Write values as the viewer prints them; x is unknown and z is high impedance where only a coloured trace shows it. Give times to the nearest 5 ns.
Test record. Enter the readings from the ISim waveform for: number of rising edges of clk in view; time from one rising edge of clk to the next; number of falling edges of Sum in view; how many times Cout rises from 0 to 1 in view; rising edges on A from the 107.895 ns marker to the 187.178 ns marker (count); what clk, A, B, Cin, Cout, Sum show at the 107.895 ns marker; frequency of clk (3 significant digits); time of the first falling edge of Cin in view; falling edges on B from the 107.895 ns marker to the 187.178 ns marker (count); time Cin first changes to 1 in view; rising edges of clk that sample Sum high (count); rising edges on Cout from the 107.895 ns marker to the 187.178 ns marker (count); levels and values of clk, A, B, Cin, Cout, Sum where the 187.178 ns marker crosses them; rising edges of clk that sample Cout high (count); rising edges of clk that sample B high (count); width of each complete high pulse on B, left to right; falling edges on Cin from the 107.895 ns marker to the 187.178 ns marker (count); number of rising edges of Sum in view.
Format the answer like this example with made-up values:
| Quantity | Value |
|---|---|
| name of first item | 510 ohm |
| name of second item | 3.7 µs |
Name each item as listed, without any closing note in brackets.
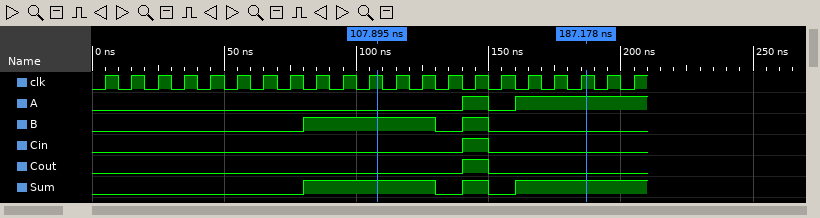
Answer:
| Quantity | Value |
|---|---|
| number of rising edges of clk in view | 21 |
| time from one rising edge of clk to the next | 10 ns |
| number of falling edges of Sum in view | 2 |
| how many times Cout rises from 0 to 1 in view | 1 |
| rising edges on A from the 107.895 ns marker to the 187.178 ns marker | 2 |
| what clk, A, B, Cin, Cout, Sum show at the 107.895 ns marker | clk=1, A=0, B=1, Cin=0, Cout=0, Sum=1 |
| frequency of clk | 100 MHz |
| time of the first falling edge of Cin in view | 150 ns |
| falling edges on B from the 107.895 ns marker to the 187.178 ns marker | 2 |
| time Cin first changes to 1 in view | 140 ns |
| rising edges of clk that sample Sum high | 11 |
| rising edges on Cout from the 107.895 ns marker to the 187.178 ns marker | 1 |
| levels and values of clk, A, B, Cin, Cout, Sum where the 187.178 ns marker crosses them | clk=1, A=1, B=0, Cin=0, Cout=0, Sum=1 |
| rising edges of clk that sample Cout high | 1 |
| rising edges of clk that sample B high | 6 |
| width of each complete high pulse on B, left to right | 50 ns, 10 ns |
| falling edges on Cin from the 107.895 ns marker to the 187.178 ns marker | 1 |
| number of rising edges of Sum in view | 3 |
